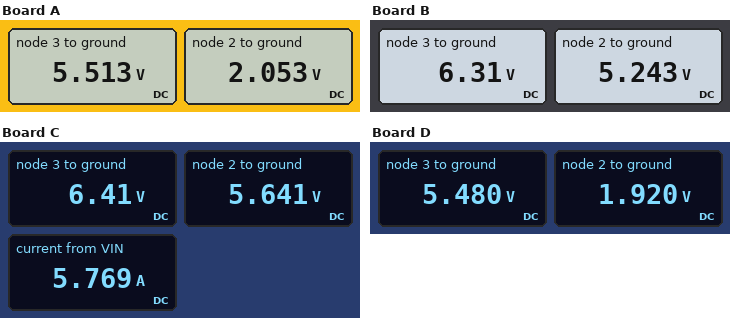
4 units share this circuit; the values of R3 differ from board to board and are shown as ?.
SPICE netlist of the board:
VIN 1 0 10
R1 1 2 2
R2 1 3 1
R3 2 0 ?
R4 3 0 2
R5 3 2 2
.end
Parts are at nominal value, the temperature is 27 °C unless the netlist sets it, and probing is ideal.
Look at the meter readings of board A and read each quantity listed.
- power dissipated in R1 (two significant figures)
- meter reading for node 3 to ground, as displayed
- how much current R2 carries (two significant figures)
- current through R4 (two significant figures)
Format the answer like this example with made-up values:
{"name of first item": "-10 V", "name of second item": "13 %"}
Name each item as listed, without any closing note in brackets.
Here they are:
{"power dissipated in R1": "32 W", "meter reading for node 3 to ground, as displayed": "5.513 V", "how much current R2 carries": "4.5 A", "current through R4": "2.8 A"}
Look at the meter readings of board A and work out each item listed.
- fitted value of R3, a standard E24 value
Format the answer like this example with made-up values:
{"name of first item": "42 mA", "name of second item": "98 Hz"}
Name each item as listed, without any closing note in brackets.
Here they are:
{"fitted value of R3, a standard E24 value": "0.36 Ω"}
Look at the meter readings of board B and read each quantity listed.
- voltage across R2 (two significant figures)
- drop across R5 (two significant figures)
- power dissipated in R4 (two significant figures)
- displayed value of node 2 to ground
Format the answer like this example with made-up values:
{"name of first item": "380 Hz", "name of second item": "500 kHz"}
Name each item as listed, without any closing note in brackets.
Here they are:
{"voltage across R2": "3.7 V", "drop across R5": "1.1 V", "power dissipated in R4": "20 W", "displayed value of node 2 to ground": "5.243 V"}
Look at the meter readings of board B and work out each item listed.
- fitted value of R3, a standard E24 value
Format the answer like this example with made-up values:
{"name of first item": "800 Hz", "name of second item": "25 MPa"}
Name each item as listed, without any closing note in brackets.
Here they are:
{"fitted value of R3, a standard E24 value": "1.8 Ω"}
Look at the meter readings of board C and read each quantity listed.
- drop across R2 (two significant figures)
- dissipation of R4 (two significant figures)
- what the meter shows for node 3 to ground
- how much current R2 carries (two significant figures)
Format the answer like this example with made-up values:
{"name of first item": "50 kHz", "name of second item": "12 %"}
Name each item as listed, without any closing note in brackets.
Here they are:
{"drop across R2": "3.6 V", "dissipation of R4": "21 W", "what the meter shows for node 3 to ground": "6.41 V", "how much current R2 carries": "3.6 A"}
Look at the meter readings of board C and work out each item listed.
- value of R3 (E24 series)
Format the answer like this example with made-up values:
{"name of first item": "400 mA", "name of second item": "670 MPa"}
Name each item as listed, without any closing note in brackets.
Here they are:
{"value of R3": "2.2 Ω"}
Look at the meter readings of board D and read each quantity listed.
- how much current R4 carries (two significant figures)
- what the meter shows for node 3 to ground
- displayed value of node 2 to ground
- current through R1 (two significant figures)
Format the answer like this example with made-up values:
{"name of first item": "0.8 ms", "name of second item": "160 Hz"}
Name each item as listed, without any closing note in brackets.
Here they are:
{"how much current R4 carries": "2.7 A", "what the meter shows for node 3 to ground": "5.480 V", "displayed value of node 2 to ground": "1.920 V", "current through R1": "4.0 A"}
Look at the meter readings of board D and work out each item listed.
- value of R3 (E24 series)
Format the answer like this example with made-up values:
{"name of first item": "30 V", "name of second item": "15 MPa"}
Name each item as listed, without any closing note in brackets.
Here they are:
{"value of R3": "0.33 Ω"}
